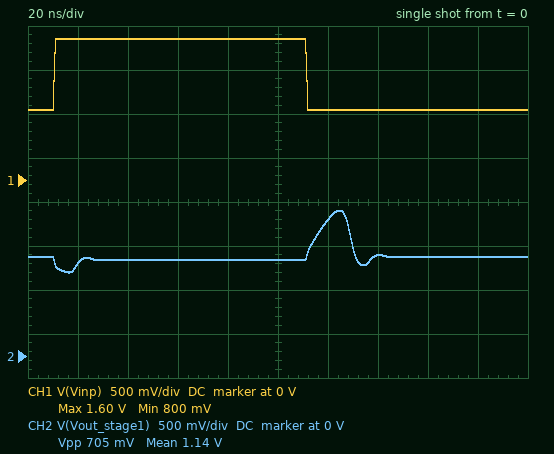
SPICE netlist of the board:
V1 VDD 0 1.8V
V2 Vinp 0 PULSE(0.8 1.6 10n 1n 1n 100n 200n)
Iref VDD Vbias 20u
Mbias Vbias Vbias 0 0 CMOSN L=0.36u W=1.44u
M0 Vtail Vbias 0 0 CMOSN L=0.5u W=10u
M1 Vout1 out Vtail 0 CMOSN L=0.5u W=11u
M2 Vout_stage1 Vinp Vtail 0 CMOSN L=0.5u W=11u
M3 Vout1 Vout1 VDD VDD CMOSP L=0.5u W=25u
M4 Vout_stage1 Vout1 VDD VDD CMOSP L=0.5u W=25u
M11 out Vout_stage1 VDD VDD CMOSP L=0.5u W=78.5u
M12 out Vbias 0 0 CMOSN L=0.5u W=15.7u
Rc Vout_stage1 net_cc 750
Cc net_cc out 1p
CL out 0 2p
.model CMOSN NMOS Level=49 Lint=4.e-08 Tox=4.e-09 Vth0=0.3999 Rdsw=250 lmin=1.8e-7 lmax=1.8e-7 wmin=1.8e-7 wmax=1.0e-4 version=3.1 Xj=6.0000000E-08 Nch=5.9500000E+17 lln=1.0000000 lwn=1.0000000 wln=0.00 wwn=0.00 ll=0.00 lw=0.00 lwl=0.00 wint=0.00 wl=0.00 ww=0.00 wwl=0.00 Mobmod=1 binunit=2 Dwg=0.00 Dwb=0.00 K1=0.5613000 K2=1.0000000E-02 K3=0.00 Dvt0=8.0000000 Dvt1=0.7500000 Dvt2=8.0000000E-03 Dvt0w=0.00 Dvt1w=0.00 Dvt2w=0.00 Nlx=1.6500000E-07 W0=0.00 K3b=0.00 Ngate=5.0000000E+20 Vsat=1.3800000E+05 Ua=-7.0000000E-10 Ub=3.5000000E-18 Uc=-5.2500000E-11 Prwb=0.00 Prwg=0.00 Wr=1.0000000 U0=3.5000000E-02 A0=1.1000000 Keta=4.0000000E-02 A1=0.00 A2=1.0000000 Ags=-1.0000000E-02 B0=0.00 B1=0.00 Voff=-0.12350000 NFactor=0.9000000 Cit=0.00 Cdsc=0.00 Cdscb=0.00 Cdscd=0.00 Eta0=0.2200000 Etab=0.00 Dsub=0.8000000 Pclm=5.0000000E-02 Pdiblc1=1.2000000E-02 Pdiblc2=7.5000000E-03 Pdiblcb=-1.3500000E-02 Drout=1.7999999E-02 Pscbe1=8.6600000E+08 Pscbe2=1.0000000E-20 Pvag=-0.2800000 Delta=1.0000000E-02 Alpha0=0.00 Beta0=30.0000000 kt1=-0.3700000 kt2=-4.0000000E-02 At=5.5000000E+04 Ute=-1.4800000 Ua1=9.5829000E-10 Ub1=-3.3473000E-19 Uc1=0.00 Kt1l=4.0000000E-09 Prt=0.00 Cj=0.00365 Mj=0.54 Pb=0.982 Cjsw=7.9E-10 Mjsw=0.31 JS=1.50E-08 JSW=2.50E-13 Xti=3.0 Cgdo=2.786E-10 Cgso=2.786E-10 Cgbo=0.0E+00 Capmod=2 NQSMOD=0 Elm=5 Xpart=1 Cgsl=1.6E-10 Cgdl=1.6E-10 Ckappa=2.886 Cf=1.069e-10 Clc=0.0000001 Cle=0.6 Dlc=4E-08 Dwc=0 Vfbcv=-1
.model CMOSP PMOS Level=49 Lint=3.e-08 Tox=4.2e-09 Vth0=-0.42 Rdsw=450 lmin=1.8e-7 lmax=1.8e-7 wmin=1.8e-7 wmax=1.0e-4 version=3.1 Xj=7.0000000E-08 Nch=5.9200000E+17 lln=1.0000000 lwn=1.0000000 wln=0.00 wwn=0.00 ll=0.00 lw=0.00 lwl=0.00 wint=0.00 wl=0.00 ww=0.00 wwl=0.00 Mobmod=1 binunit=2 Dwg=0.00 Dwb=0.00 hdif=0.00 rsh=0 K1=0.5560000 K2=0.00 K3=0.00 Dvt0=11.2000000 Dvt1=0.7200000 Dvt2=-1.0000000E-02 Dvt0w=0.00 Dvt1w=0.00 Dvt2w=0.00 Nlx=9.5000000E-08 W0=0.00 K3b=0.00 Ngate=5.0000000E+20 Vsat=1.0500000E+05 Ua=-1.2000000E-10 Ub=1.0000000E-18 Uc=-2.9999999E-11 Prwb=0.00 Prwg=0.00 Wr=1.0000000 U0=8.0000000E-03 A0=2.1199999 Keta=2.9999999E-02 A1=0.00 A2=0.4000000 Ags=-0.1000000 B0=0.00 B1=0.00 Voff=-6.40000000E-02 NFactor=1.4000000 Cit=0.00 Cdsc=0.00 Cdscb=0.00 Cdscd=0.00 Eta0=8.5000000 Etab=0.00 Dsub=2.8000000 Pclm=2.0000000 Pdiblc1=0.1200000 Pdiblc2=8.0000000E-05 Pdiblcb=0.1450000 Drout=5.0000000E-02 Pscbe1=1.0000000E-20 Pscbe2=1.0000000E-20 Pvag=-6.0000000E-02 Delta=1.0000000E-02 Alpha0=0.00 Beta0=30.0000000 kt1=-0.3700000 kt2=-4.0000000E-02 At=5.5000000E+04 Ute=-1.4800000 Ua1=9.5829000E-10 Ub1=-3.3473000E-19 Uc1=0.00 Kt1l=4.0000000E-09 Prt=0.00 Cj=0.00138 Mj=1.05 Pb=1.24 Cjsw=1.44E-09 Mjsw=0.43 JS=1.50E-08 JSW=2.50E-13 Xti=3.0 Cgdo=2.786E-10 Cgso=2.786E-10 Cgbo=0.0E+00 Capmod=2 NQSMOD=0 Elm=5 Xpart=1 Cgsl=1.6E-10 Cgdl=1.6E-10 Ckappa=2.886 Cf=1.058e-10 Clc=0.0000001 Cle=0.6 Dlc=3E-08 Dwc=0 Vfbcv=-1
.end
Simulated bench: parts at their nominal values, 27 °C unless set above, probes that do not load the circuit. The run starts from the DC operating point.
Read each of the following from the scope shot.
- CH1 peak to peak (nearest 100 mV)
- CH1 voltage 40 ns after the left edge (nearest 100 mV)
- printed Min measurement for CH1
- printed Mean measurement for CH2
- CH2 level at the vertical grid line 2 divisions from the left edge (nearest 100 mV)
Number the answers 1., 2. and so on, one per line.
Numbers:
1. 800 mV
2. 1.6 V
3. 800 mV
4. 1.14 V
5. 1.1 V
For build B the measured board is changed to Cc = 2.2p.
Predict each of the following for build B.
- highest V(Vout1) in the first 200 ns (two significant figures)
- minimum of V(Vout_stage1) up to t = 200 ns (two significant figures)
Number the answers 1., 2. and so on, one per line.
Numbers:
1. 1.4 V
2. 1.0 V
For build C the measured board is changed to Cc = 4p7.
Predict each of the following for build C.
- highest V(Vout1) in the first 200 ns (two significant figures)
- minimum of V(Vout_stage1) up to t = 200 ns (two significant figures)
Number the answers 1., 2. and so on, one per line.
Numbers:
1. 1.4 V
2. 1.0 V
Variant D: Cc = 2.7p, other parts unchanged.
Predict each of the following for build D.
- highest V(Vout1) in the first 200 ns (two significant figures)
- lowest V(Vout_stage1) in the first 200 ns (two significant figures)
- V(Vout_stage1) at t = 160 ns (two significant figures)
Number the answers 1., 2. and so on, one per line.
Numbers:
1. 1.4 V
2. 1.0 V
3. 1.1 V
